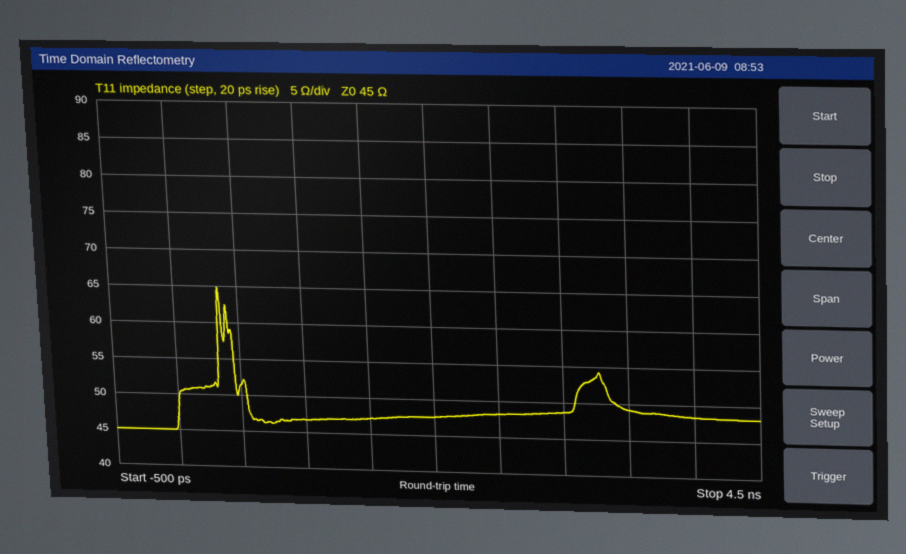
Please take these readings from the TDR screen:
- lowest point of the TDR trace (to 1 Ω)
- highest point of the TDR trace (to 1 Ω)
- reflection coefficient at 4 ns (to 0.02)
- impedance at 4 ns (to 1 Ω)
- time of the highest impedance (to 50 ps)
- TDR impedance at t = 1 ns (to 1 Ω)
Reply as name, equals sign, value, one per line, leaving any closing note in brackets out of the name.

lowest point of the TDR trace = 45 Ω
highest point of the TDR trace = 65 Ω
reflection coefficient at 4 ns = +0.04
impedance at 4 ns = 48 Ω
time of the highest impedance = 350 ps
TDR impedance at t = 1 ns = 47 Ω
